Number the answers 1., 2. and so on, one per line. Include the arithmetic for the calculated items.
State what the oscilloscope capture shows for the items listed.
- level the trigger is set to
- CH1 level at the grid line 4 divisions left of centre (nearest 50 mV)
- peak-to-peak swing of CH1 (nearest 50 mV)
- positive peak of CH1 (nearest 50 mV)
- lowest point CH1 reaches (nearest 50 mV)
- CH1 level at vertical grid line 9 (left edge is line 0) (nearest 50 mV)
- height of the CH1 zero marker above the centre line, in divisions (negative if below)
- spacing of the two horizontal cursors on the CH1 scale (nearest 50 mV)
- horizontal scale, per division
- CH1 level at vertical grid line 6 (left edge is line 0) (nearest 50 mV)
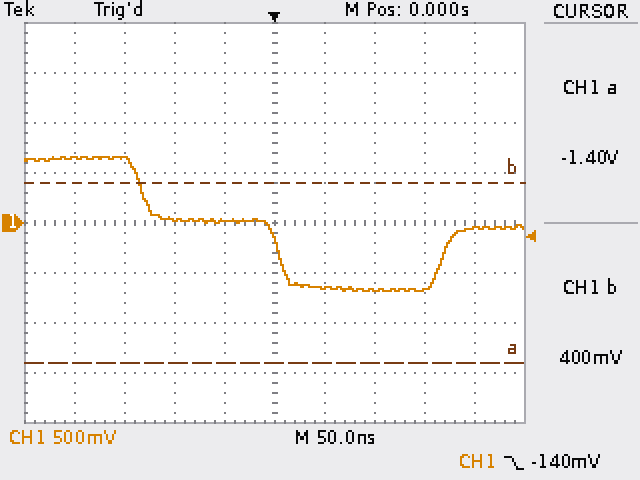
1. -140 mV
2. 650 mV
3. 650 mV − (-700 mV) = 1.35 V
4. 650 mV
5. -700 mV
6. -50 mV
7. 0.0 div
8. 1.80 V
9. 50 ns
10. -650 mV
